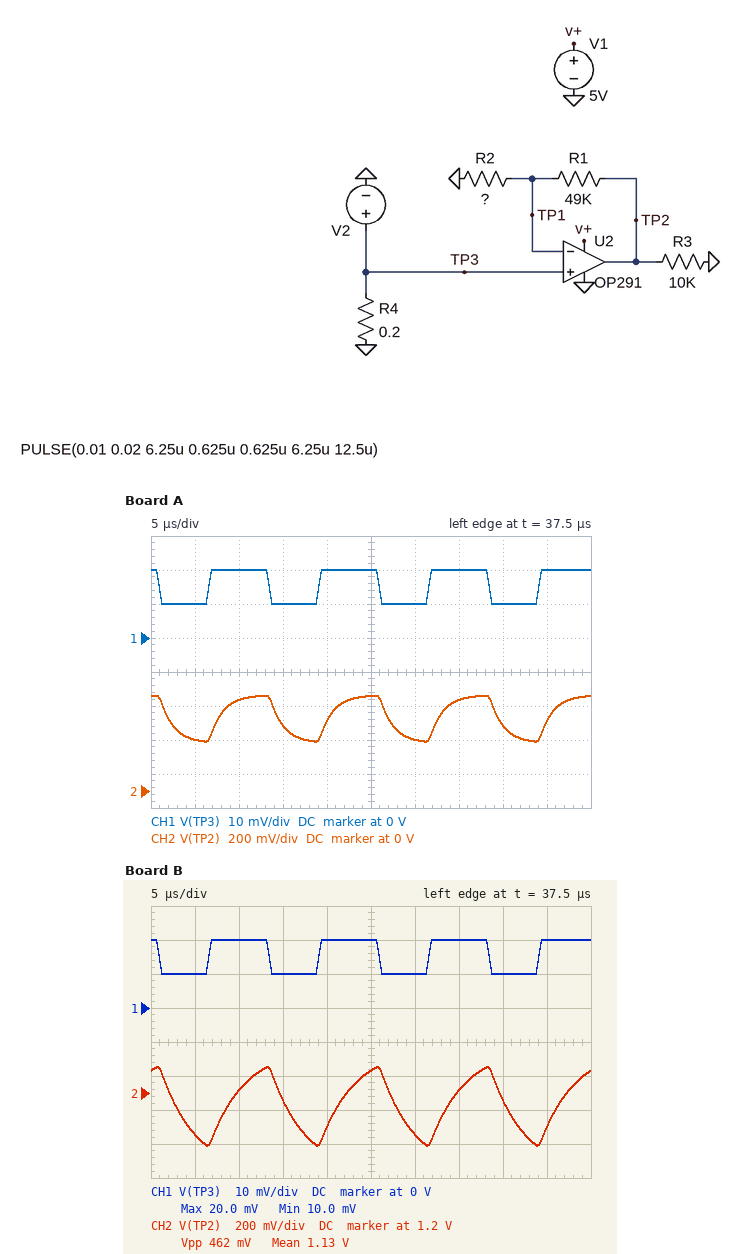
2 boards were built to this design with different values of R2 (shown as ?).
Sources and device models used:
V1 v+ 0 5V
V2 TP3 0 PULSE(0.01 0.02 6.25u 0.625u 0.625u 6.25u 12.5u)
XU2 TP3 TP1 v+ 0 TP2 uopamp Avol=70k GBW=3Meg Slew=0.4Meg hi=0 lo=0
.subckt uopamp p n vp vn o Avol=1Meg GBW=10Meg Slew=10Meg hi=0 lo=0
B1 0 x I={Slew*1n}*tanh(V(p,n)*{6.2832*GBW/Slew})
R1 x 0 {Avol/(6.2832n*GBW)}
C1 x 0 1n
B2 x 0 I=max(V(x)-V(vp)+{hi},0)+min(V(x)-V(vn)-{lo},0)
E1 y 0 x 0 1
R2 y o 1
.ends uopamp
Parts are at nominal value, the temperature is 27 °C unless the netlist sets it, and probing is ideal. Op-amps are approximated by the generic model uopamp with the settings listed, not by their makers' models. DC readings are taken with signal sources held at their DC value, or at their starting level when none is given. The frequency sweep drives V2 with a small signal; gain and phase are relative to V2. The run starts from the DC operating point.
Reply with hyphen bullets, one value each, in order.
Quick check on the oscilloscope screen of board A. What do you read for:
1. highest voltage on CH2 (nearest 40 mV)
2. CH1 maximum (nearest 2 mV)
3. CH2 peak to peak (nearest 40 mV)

- 560 mV
- 20 mV
- 280 mV
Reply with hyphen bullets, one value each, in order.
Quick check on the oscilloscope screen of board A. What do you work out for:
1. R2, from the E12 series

- 1.8 kΩ
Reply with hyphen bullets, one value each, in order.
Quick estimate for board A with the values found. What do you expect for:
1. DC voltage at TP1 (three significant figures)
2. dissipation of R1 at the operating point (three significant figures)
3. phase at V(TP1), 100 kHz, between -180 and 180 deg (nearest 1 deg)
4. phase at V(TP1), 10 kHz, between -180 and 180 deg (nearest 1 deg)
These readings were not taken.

- 10.0 mV
- 1.51 µW
- -43 deg
- -5 deg
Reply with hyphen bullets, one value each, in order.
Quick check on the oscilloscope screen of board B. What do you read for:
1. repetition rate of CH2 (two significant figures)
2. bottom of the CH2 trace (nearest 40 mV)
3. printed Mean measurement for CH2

- 80 kHz
- 880 mV
- 1.13 V
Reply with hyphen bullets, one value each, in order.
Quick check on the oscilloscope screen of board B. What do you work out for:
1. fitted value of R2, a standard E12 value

- 680 Ω
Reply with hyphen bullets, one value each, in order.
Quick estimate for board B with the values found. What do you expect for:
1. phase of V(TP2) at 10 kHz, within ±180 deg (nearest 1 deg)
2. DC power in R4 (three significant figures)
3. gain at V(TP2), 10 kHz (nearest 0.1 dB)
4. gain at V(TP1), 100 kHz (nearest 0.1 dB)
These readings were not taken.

- -14 deg
- 500 µW
- 37.0 dB
- -8.4 dB
